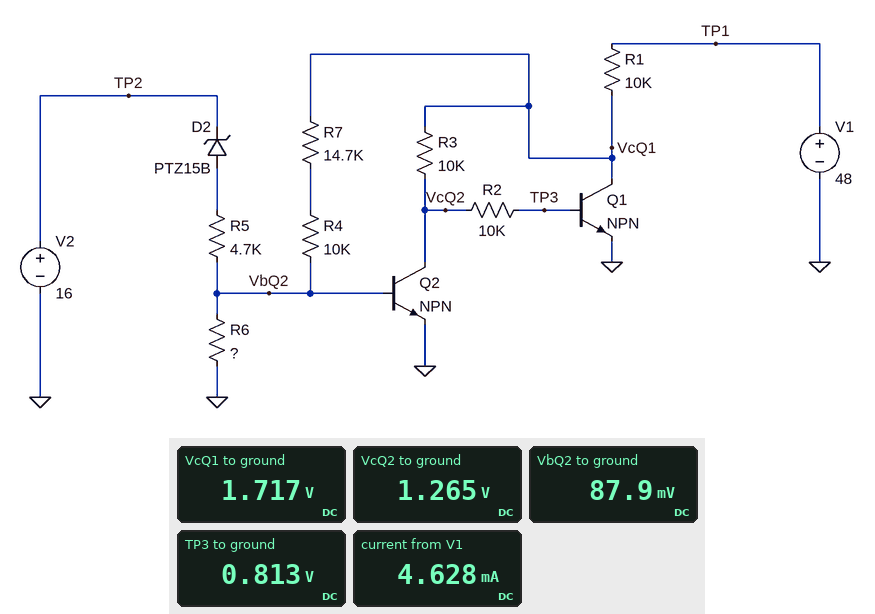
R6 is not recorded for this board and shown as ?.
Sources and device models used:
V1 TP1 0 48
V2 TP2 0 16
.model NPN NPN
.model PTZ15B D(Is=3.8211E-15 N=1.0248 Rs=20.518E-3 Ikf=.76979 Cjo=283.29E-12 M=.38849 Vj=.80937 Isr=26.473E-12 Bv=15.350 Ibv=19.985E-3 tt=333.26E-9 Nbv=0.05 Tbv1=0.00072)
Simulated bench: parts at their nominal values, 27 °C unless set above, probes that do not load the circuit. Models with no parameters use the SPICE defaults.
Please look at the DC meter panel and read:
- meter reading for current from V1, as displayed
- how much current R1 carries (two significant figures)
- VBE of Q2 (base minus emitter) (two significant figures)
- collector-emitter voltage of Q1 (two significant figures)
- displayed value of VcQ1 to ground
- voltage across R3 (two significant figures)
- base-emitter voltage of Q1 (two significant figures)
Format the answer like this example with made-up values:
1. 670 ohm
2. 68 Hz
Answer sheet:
1. 4.628 mA
2. 4.6 mA
3. 88 mV
4. 1.7 V
5. 1.717 V
6. 450 mV
7. 810 mV
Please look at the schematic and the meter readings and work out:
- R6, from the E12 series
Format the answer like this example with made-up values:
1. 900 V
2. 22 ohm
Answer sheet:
1. 470 Ω
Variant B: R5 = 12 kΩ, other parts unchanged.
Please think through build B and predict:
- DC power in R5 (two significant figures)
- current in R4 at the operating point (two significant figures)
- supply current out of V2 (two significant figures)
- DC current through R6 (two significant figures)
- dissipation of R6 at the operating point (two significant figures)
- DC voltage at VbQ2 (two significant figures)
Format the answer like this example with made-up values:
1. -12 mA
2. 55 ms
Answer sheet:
1. 30 µW
2. 67 µA
3. 50 µA
4. 120 µA
5. 6.5 µW
6. 55 mV
